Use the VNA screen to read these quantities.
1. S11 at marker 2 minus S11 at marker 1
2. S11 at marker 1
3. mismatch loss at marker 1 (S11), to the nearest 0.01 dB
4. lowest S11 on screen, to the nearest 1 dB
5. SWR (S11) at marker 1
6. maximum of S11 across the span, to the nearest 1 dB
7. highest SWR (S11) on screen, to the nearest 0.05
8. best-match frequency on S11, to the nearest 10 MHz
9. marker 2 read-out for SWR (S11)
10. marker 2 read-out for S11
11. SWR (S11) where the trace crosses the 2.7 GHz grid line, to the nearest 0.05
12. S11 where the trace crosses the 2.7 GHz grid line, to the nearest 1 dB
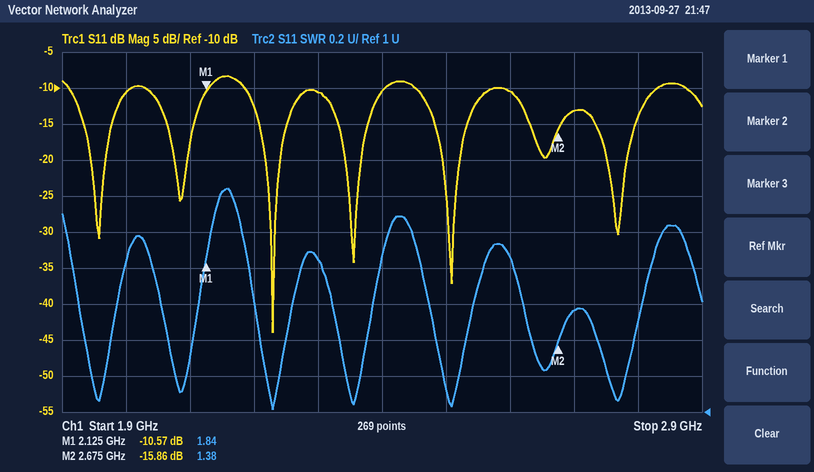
-5.29 dB
-10.57 dB
0.40 dB
-44 dB
1.84
-8 dB
2.25
2.23 GHz
1.38
-15.86 dB
1.55
-13 dB
